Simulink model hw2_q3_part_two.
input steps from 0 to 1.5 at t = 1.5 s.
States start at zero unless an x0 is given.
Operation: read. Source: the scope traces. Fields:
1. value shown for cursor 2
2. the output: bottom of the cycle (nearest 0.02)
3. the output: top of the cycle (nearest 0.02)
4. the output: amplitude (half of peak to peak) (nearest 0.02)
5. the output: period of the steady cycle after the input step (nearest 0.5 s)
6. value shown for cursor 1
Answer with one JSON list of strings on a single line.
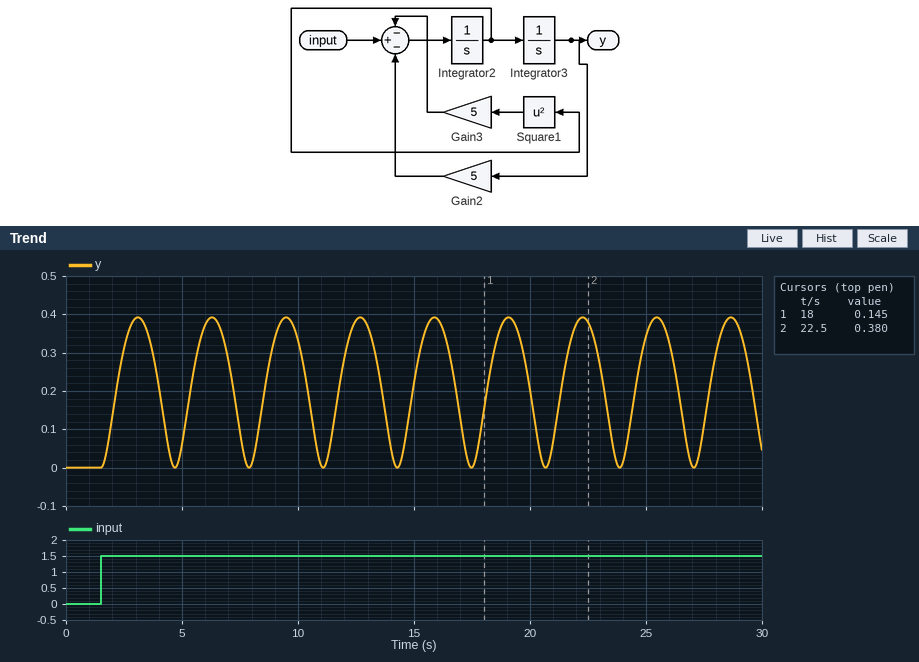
["0.380", "0.00", "0.40", "0.20", "3.0 s", "0.145"]
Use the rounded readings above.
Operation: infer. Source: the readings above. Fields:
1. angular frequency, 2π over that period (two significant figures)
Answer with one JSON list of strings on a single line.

["2.1 rad/s"]
